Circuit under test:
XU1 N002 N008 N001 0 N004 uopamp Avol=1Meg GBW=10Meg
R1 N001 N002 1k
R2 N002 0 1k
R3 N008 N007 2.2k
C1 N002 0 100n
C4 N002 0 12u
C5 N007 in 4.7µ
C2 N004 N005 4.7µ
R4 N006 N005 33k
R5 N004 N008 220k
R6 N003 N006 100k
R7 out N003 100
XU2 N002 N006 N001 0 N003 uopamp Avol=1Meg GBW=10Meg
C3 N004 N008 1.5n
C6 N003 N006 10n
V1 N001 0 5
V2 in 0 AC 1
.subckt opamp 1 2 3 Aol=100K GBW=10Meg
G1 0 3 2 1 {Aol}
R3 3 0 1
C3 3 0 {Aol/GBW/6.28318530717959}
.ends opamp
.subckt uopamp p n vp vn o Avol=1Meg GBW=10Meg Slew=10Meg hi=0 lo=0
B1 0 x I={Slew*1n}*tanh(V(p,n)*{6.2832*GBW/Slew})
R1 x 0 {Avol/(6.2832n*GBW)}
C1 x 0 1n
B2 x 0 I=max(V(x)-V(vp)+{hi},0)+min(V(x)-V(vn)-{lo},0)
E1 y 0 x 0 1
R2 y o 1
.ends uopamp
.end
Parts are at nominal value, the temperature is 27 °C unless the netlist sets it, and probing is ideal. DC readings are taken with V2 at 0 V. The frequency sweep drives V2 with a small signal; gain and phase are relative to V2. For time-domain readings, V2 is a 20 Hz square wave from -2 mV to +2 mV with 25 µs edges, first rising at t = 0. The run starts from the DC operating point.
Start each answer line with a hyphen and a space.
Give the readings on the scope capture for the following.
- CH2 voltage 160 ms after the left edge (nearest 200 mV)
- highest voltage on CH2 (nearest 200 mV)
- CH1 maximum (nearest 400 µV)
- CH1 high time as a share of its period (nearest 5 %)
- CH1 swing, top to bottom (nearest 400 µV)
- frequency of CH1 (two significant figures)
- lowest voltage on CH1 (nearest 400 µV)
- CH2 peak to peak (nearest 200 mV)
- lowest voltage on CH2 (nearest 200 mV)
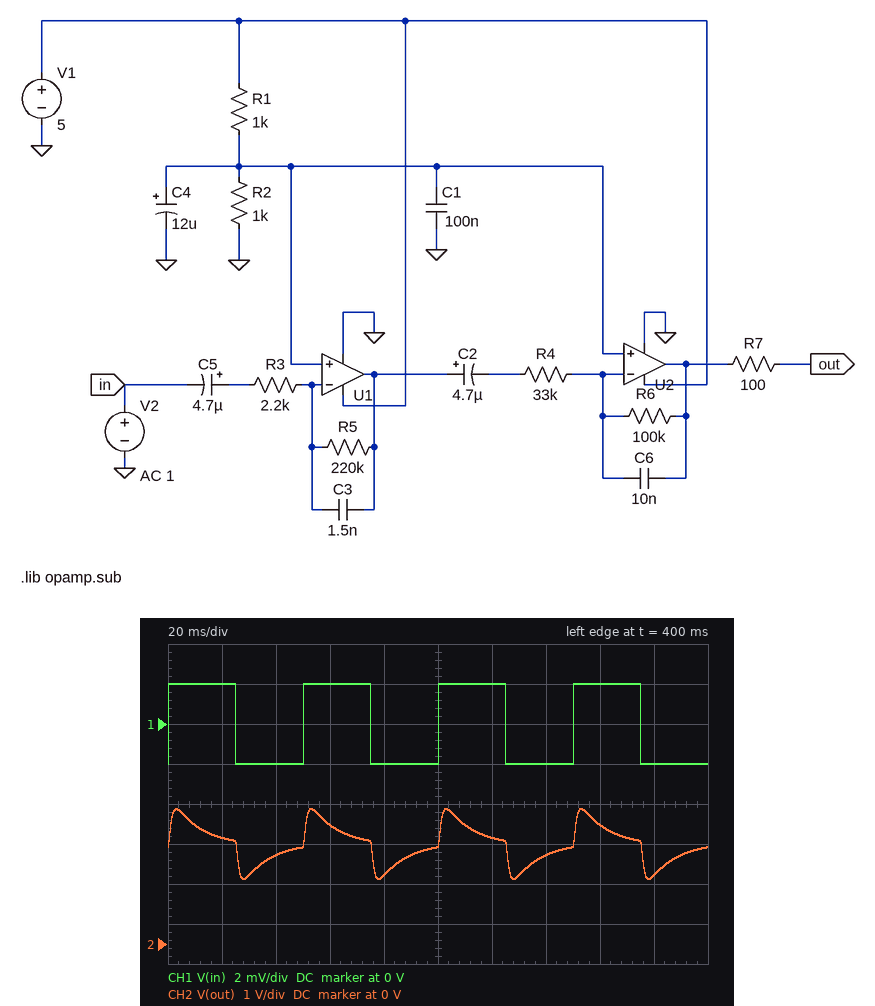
- 3.0 V
- 3.4 V
- 2.0 mV
- 50 %
- 4.0 mV
- 20 Hz
- -2.0 mV
- 1.8 V
- 1.6 V
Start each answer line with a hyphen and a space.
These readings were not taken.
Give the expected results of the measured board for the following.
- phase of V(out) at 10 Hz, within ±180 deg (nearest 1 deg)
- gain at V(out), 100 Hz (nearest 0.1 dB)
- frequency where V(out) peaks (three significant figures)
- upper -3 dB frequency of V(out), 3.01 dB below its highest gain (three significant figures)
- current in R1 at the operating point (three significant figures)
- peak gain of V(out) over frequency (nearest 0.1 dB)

- 58 deg
- 47.9 dB
- 48.1 Hz
- 170 Hz
- 2.50 mA
- 48.8 dB
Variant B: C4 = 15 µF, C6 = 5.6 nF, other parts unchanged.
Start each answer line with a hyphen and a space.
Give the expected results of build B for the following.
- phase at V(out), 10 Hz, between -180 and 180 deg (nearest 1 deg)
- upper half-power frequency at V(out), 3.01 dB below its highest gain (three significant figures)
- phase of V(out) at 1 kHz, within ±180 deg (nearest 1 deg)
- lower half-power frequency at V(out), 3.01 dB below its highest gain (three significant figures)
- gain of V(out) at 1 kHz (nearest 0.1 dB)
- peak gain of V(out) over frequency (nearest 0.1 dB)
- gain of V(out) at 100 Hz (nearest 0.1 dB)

- 60 deg
- 250 Hz
- -138 deg
- 13.8 Hz
- 31.1 dB
- 49.1 dB
- 48.8 dB
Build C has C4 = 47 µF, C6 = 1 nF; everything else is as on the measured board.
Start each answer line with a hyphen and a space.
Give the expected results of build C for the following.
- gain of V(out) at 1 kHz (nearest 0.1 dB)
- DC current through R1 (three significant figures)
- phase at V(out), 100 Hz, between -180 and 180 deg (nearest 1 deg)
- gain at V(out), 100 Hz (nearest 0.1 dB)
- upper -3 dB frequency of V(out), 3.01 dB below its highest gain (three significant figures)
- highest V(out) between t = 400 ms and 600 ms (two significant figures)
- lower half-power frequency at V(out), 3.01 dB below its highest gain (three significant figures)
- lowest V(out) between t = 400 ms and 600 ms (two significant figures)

- 40.9 dB
- 2.50 mA
- -6 deg
- 49.3 dB
- 471 Hz
- 3.5 V
- 14.5 Hz
- 1.5 V
